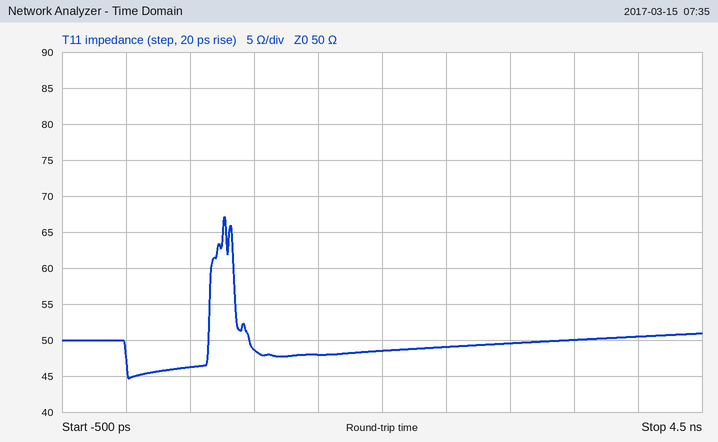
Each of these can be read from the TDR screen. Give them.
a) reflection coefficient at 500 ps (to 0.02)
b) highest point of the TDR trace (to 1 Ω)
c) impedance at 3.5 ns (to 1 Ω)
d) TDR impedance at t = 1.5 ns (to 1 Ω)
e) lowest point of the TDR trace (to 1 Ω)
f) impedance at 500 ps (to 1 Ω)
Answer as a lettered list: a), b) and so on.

a) -0.04
b) 67 Ω
c) 50 Ω
d) 48 Ω
e) 45 Ω
f) 46 Ω
